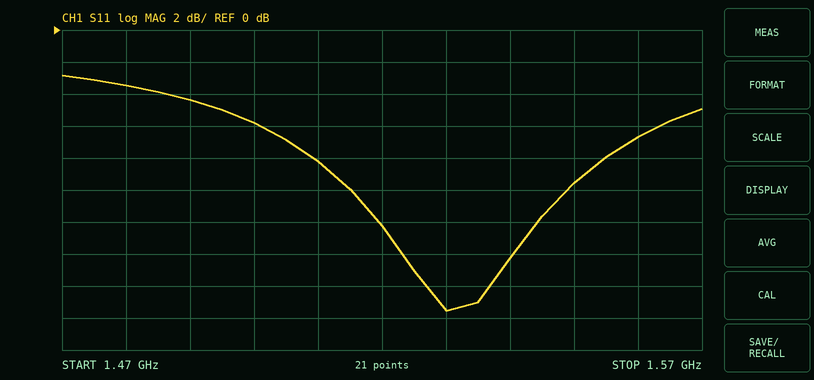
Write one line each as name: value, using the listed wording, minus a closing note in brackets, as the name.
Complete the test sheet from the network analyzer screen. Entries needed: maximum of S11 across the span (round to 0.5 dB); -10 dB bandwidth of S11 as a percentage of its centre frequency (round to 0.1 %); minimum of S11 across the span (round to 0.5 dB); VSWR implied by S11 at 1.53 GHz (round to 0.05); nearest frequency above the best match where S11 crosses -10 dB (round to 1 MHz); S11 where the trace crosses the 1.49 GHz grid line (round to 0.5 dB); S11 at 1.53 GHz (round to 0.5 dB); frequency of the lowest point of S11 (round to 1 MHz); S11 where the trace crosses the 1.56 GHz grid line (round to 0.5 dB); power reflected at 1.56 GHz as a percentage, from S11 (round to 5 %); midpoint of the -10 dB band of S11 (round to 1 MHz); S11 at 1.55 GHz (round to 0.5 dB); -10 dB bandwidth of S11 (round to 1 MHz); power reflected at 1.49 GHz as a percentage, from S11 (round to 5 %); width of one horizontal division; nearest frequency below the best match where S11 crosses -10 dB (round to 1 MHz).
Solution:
maximum of S11 across the span: -3.0 dB
-10 dB bandwidth of S11 as a percentage of its centre frequency: 2.2 %
minimum of S11 across the span: -17.5 dB
VSWR implied by S11 at 1.53 GHz: 1.30
nearest frequency above the best match where S11 crosses -10 dB: 1.549 GHz
S11 where the trace crosses the 1.49 GHz grid line: -4.5 dB
S11 at 1.53 GHz: -17.5 dB
frequency of the lowest point of S11: 1.530 GHz
S11 where the trace crosses the 1.56 GHz grid line: -6.5 dB
power reflected at 1.56 GHz as a percentage, from S11: 20 %
midpoint of the -10 dB band of S11: 1.532 GHz
S11 at 1.55 GHz: -9.5 dB
-10 dB bandwidth of S11: 34 MHz
power reflected at 1.49 GHz as a percentage, from S11: 35 %
width of one horizontal division: 10 MHz
nearest frequency below the best match where S11 crosses -10 dB: 1.515 GHz
